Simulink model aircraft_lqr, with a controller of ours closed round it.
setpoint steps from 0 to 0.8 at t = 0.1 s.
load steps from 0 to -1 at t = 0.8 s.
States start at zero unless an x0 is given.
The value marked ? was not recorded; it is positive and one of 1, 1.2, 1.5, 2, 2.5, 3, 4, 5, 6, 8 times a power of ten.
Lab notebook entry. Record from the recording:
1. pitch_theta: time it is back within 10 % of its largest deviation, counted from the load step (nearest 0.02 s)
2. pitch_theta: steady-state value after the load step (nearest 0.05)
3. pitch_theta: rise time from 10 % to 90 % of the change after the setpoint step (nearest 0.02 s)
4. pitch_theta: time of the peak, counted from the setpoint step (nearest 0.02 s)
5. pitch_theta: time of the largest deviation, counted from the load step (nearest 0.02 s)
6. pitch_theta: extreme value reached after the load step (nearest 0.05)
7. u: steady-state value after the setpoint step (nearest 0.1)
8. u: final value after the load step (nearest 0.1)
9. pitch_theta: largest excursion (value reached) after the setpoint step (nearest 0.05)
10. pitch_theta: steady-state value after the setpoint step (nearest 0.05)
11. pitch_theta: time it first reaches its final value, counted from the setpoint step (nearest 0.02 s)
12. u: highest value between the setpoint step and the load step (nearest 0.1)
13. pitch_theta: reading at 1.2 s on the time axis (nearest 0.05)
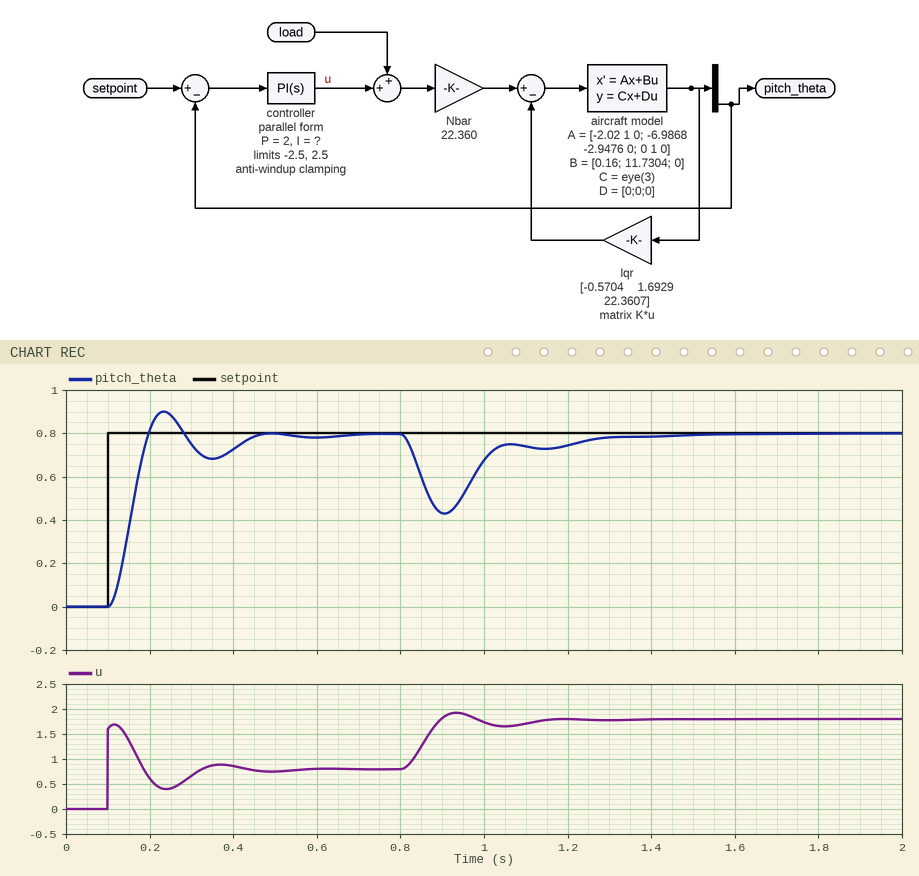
0.44 s
0.80
0.06 s
0.14 s
0.10 s
0.45
0.8
1.8
0.90
0.80
0.10 s
1.7
0.75
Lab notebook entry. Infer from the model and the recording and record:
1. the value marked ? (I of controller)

15
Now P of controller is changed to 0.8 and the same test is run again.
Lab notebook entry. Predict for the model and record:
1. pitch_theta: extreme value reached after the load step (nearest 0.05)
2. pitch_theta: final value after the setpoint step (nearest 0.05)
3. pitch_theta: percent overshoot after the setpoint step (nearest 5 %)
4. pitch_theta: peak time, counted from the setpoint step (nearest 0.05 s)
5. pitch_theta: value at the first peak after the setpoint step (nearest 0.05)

0.30
0.80
20 %
0.20 s
0.95
